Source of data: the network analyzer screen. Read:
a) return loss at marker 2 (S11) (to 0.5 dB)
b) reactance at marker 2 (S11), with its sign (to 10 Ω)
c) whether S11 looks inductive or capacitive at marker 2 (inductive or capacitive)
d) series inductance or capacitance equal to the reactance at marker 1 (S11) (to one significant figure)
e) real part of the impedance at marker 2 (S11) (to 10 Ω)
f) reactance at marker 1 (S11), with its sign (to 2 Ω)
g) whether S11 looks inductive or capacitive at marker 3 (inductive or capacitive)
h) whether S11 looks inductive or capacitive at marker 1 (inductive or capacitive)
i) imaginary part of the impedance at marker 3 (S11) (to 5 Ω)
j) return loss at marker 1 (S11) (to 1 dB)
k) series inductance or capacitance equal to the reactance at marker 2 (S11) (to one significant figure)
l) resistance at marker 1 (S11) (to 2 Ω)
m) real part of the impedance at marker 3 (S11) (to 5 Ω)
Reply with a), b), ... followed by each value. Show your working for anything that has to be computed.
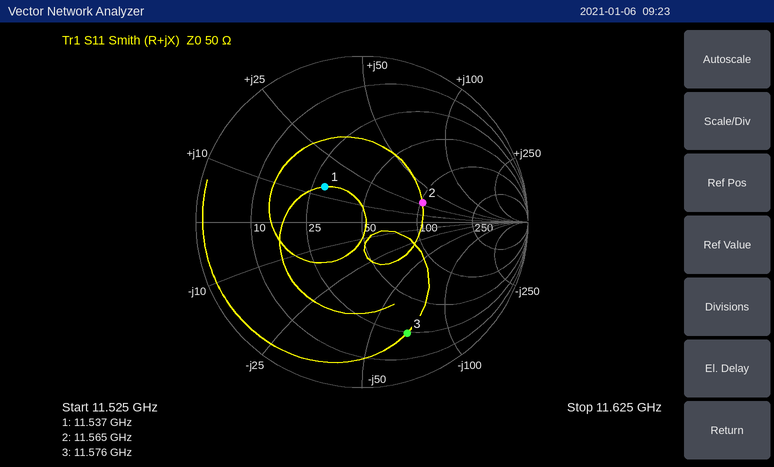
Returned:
a) 8.5 dB
b) +30 Ω
c) inductive
d) L = 14 Ω/(2π × 11.537 GHz) ≈ 193 pH, so 200 pH to one significant figure
e) 100 Ω
f) +14 Ω
g) capacitive
h) inductive
i) -70 Ω
j) 10 dB
k) L = 30 Ω/(2π × 11.565 GHz) ≈ 413 pH, so 400 pH to one significant figure
l) 30 Ω
m) 25 Ω
